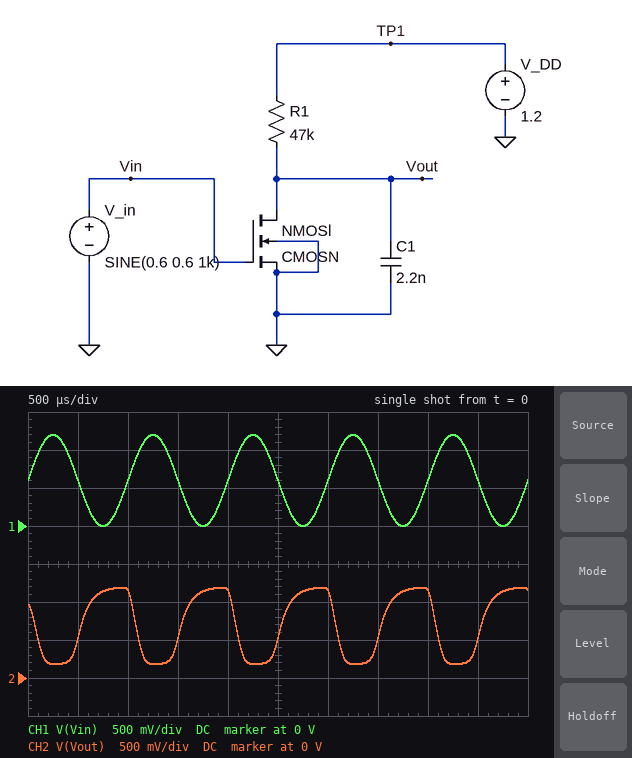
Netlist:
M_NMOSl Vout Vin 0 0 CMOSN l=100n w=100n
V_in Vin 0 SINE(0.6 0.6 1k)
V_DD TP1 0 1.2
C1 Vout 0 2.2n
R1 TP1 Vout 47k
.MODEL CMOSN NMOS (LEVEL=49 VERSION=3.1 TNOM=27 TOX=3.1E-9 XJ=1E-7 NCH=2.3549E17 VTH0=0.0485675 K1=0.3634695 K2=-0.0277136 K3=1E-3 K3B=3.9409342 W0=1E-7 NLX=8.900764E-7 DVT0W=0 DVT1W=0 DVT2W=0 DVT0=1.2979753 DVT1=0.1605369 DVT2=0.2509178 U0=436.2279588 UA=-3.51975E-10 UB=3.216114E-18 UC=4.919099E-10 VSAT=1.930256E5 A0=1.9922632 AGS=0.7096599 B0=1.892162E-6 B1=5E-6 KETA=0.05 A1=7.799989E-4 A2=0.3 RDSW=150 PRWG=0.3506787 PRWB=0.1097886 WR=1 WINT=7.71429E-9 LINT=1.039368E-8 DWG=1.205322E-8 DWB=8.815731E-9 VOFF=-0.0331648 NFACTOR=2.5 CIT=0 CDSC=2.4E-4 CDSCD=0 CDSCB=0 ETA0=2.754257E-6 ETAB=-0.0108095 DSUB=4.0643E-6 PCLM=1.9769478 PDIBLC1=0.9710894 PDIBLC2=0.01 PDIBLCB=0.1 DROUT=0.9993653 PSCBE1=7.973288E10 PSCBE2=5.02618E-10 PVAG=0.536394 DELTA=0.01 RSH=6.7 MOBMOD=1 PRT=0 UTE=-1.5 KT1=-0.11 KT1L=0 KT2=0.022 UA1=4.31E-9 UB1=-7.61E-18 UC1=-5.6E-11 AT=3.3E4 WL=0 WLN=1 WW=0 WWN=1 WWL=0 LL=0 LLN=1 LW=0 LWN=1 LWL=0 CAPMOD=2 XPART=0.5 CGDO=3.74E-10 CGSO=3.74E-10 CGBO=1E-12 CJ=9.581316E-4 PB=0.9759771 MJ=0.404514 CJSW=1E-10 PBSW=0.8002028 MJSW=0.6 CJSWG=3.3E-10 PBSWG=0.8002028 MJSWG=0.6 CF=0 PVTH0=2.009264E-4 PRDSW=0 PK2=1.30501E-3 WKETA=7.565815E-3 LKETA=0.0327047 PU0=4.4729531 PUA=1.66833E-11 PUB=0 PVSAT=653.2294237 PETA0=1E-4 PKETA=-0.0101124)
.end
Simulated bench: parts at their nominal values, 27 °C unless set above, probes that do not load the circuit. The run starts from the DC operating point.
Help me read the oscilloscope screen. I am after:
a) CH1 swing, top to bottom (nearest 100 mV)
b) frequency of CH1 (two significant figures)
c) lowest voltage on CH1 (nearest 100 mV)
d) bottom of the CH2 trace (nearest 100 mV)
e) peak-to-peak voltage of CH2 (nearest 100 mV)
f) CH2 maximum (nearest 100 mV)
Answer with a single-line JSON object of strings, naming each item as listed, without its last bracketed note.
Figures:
{"CH1 swing, top to bottom": "1.2 V", "frequency of CH1": "1.0 kHz", "lowest voltage on CH1": "0 V", "bottom of the CH2 trace": "200 mV", "peak-to-peak voltage of CH2": "1.0 V", "CH2 maximum": "1.2 V"}
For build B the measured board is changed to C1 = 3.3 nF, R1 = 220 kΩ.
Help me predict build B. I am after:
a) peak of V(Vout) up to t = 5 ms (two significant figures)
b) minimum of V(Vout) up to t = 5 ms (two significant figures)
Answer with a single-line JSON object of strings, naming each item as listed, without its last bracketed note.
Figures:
{"peak of V(Vout) up to t = 5 ms": "630 mV", "minimum of V(Vout) up to t = 5 ms": "38 mV"}
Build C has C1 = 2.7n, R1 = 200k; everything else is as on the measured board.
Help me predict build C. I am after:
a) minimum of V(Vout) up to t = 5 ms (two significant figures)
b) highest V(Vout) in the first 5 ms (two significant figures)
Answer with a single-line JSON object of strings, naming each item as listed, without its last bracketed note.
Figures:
{"minimum of V(Vout) up to t = 5 ms": "42 mV", "highest V(Vout) in the first 5 ms": "750 mV"}
